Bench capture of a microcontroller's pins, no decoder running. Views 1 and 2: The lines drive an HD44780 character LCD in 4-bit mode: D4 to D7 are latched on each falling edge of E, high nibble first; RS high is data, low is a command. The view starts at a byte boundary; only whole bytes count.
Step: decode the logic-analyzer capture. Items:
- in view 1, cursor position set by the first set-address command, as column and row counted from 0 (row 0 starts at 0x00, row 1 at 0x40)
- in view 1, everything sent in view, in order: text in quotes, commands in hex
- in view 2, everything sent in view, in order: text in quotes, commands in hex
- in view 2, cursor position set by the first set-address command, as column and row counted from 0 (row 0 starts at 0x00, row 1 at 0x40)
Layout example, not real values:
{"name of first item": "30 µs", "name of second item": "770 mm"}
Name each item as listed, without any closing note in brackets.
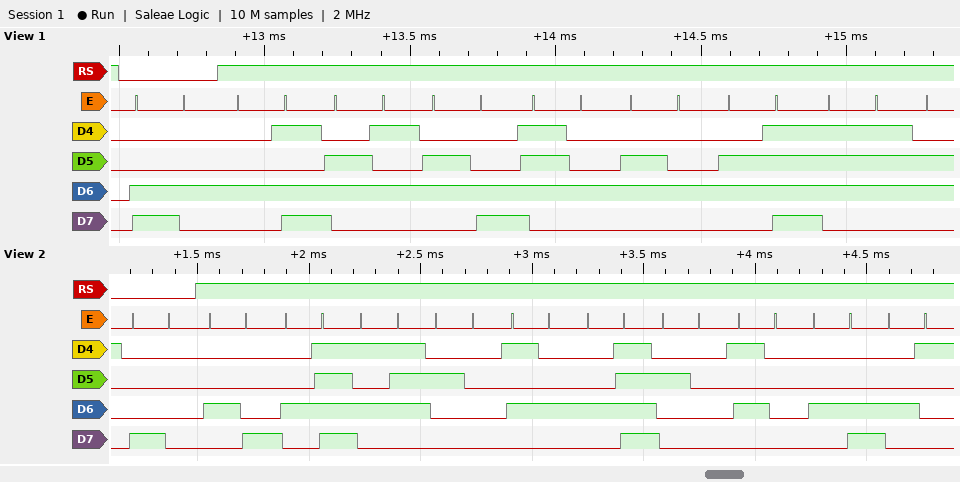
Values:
{"in view 1, cursor position set by the first set-address command, as column and row counted from 0": "column 4, row 1", "in view 1, everything sent in view, in order: text in quotes, commands in hex": "0xC4 \"Meltdow\"", "in view 2, everything sent in view, in order: text in quotes, commands in hex": "0x80 \"HOW TO PLA\"", "in view 2, cursor position set by the first set-address command, as column and row counted from 0": "column 0, row 0"}
